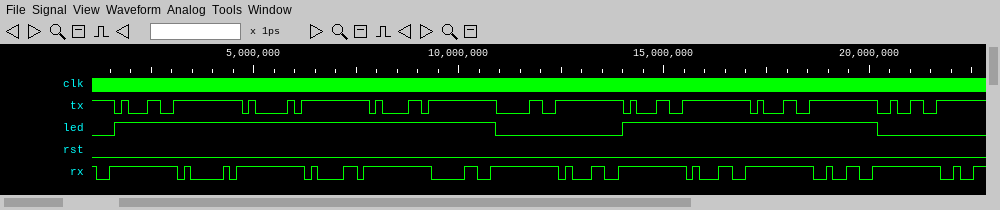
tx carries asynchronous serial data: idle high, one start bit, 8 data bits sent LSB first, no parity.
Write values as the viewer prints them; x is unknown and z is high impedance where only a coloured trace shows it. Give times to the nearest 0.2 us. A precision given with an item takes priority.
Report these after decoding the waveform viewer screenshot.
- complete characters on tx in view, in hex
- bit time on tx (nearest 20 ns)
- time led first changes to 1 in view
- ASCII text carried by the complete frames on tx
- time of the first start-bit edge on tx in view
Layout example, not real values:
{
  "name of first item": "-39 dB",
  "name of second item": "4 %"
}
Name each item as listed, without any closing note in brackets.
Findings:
{
  "complete characters on tx in view, in hex": "31, 41, 61, 30, 31, 31, 32",
  "bit time on tx": "160 ns",
  "time led first changes to 1 in view": "1.6 us",
  "ASCII text carried by the complete frames on tx": "\"1Aa0112\"",
  "time of the first start-bit edge on tx in view": "1.6 us"
}
